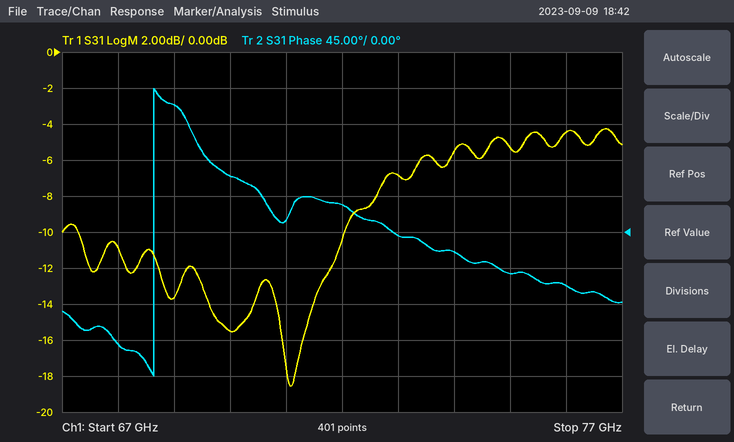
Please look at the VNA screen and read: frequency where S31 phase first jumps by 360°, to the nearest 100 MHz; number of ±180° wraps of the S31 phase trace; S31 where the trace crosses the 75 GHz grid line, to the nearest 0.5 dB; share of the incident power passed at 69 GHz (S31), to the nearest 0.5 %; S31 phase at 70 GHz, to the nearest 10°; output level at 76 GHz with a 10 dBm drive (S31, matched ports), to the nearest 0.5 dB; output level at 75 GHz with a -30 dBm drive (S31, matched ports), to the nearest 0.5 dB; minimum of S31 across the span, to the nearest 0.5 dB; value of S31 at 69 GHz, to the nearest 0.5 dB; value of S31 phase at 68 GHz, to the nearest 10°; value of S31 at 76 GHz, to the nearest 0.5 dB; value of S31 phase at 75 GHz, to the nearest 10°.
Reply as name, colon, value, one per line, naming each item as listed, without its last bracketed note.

frequency where S31 phase first jumps by 360°, to the nearest 100 MHz: 68.6 GHz
number of ±180° wraps of the S31 phase trace: 1
S31 where the trace crosses the 75 GHz grid line, to the nearest 0.5 dB: -5.5 dB
share of the incident power passed at 69 GHz (S31), to the nearest 0.5 %: 4.5 %
S31 phase at 70 GHz, to the nearest 10°: 70°
output level at 76 GHz with a 10 dBm drive (S31, matched ports), to the nearest 0.5 dB: 5.5 dBm
output level at 75 GHz with a -30 dBm drive (S31, matched ports), to the nearest 0.5 dB: -35.5 dBm
minimum of S31 across the span, to the nearest 0.5 dB: -18.5 dB
value of S31 at 69 GHz, to the nearest 0.5 dB: -13.5 dB
value of S31 phase at 68 GHz, to the nearest 10°: -140°
value of S31 at 76 GHz, to the nearest 0.5 dB: -4.5 dB
value of S31 phase at 75 GHz, to the nearest 10°: -50°
